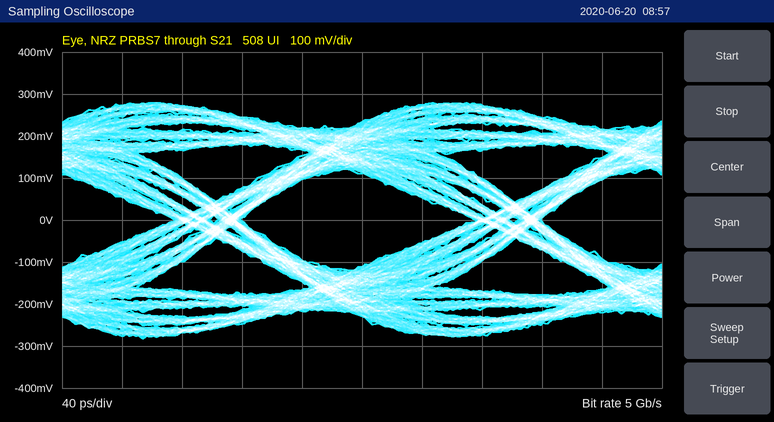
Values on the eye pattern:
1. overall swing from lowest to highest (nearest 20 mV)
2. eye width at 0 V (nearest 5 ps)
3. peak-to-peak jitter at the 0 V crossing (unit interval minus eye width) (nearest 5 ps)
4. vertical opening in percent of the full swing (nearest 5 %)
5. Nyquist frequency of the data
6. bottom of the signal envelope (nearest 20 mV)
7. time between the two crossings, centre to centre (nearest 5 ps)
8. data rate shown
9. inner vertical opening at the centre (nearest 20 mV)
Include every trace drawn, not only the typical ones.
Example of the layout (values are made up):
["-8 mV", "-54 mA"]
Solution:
["560 mV", "155 ps", "45 ps", "40 %", "2.5 GHz", "-280 mV", "200 ps", "5 Gb/s", "220 mV"]
